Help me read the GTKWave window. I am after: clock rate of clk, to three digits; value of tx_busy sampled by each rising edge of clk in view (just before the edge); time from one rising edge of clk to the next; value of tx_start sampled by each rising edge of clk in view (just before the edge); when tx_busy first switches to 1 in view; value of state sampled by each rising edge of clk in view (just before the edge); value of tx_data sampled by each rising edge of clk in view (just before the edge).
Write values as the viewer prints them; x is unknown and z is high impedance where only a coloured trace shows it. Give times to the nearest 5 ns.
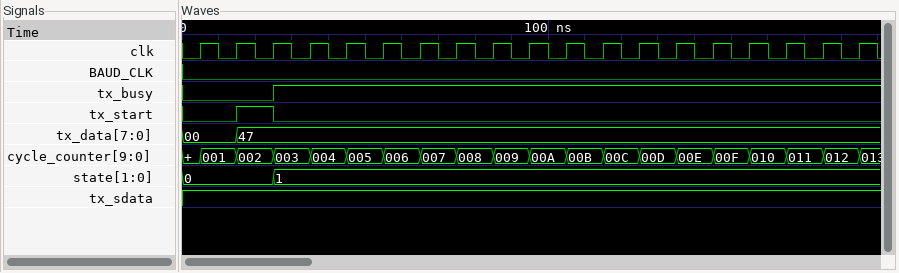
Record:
100 MHz
0 0 0 1 1 1 1 1 1 1 1 1 1 1 1 1 1 1 1
10 ns
0 0 1 0 0 0 0 0 0 0 0 0 0 0 0 0 0 0 0
25 ns
0, 0, 0, 1, 1, 1, 1, 1, 1, 1, 1, 1, 1, 1, 1, 1, 1, 1, 1
00, 00, 47, 47, 47, 47, 47, 47, 47, 47, 47, 47, 47, 47, 47, 47, 47, 47, 47
